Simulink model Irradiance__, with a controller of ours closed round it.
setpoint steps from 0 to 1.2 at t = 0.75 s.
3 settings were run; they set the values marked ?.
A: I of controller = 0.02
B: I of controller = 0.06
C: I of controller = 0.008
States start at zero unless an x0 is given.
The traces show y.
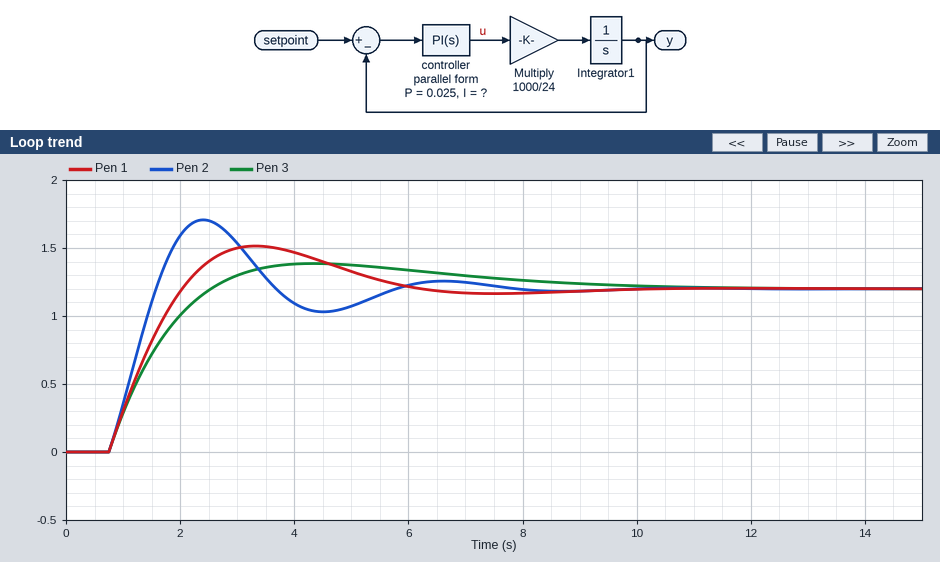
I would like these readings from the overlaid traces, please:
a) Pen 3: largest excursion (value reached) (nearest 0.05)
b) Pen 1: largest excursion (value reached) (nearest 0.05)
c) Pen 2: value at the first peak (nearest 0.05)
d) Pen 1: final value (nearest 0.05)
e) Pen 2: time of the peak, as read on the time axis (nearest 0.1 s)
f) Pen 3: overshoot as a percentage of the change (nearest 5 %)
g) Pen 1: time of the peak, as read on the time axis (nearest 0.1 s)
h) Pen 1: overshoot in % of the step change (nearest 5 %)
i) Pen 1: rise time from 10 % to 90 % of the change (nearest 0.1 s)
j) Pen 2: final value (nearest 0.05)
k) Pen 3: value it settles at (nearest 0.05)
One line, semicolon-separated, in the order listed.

1.40; 1.50; 1.70; 1.20; 2.4 s; 15 %; 3.3 s; 25 %; 1.0 s; 1.20; 1.20
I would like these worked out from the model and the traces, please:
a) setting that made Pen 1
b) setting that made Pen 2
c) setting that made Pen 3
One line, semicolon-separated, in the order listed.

A; B; C
